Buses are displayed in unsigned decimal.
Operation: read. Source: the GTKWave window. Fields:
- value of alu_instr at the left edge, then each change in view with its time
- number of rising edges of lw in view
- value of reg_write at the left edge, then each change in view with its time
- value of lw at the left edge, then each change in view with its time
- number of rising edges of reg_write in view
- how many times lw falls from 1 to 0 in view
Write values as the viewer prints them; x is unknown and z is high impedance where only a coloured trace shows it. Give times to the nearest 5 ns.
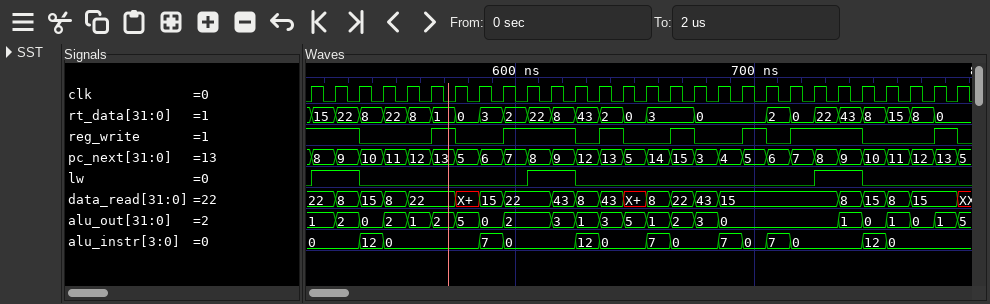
0, 12 at 535 ns, 0 at 545 ns, 7 at 585 ns, 0 at 595 ns, 12 at 625 ns, 0 at 635 ns, 7 at 655 ns, 0 at 665 ns, 7 at 685 ns, 0 at 695 ns, 7 at 705 ns, 0 at 715 ns, 12 at 745 ns, 0 at 755 ns
3
1, 0 at 535 ns, 1 at 565 ns, 0 at 575 ns, 1 at 595 ns, 0 at 625 ns, 1 at 635 ns, 0 at 645 ns, 1 at 665 ns, 0 at 675 ns, 1 at 695 ns, 0 at 705 ns, 1 at 715 ns, 0 at 745 ns, 1 at 775 ns, 0 at 785 ns
0, 1 at 515 ns, 0 at 535 ns, 1 at 605 ns, 0 at 625 ns, 1 at 725 ns, 0 at 745 ns
7
3
